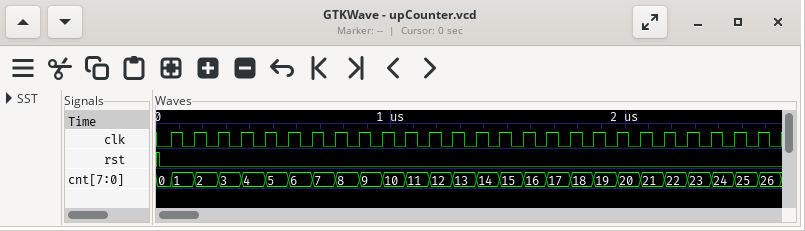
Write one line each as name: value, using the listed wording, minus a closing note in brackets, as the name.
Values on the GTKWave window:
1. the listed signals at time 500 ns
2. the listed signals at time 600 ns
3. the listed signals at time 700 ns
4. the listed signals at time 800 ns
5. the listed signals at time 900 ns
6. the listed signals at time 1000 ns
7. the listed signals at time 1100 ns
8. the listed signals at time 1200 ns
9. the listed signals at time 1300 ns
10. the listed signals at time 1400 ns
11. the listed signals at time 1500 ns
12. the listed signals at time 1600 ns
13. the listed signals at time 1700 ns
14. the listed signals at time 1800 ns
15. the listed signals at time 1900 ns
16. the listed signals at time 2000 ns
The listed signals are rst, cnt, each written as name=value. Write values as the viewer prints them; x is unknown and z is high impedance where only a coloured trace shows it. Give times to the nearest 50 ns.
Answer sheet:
the listed signals at time 500 ns: rst=0, cnt=5
the listed signals at time 600 ns: rst=0, cnt=6
the listed signals at time 700 ns: rst=0, cnt=7
the listed signals at time 800 ns: rst=0, cnt=8
the listed signals at time 900 ns: rst=0, cnt=9
the listed signals at time 1000 ns: rst=0, cnt=10
the listed signals at time 1100 ns: rst=0, cnt=11
the listed signals at time 1200 ns: rst=0, cnt=12
the listed signals at time 1300 ns: rst=0, cnt=13
the listed signals at time 1400 ns: rst=0, cnt=14
the listed signals at time 1500 ns: rst=0, cnt=15
the listed signals at time 1600 ns: rst=0, cnt=16
the listed signals at time 1700 ns: rst=0, cnt=17
the listed signals at time 1800 ns: rst=0, cnt=18
the listed signals at time 1900 ns: rst=0, cnt=19
the listed signals at time 2000 ns: rst=0, cnt=20
